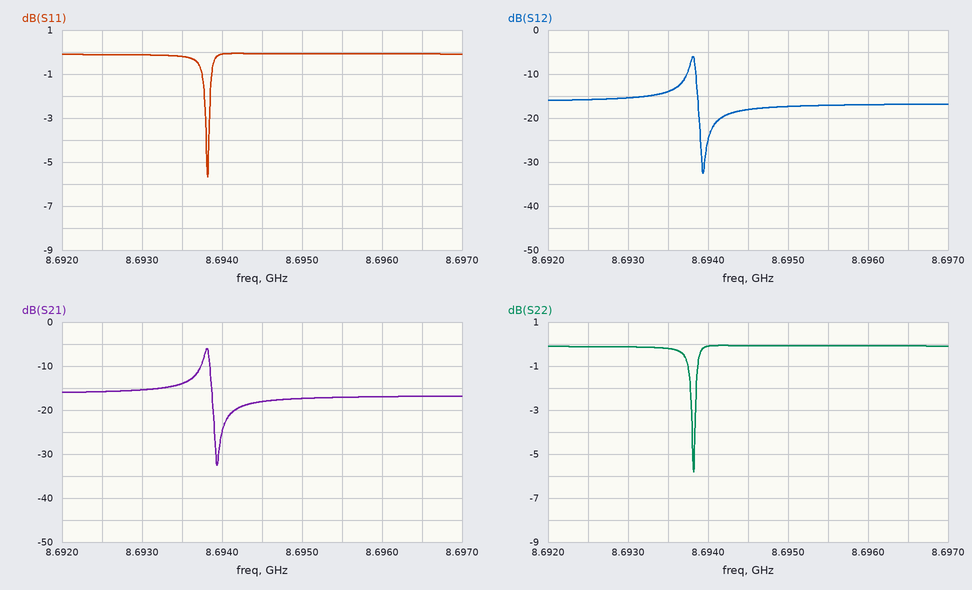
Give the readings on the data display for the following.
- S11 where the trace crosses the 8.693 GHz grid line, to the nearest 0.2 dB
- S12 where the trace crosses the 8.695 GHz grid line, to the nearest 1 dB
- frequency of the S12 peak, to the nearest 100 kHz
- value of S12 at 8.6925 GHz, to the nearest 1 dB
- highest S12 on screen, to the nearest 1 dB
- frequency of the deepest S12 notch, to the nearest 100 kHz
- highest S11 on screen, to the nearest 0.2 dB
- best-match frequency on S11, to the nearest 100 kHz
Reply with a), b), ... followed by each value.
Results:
a) -0.2 dB
b) -17 dB
c) 8.6938 GHz
d) -16 dB
e) -6 dB
f) 8.6939 GHz
g) 0.0 dB
h) 8.6938 GHz
